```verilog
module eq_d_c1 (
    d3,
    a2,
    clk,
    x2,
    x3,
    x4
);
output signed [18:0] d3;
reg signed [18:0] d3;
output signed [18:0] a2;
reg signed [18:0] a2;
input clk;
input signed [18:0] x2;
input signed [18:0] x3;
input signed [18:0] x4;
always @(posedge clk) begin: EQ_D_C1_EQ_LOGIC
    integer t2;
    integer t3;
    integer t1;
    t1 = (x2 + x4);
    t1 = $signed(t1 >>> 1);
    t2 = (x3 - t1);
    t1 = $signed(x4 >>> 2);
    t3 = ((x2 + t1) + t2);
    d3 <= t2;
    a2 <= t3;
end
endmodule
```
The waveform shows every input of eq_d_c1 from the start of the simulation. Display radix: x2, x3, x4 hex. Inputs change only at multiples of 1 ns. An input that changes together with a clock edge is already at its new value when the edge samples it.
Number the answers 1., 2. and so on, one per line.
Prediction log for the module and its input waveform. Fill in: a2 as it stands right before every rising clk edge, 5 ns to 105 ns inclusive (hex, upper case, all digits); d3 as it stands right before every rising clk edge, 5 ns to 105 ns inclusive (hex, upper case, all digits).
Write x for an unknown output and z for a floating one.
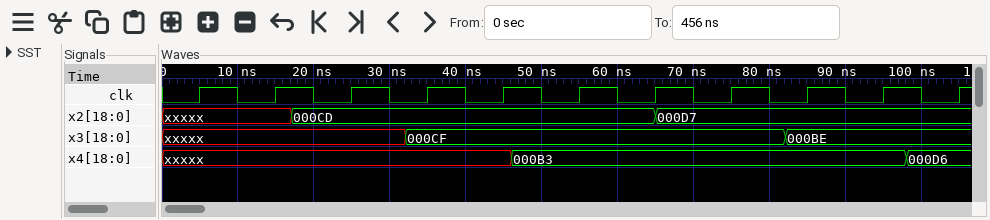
1. x, x, x, x, x, x, 00108, 0010D, 0010D, 000FC, 000FC
2. x, x, x, x, x, x, 0000F, 0000A, 0000A, 7FFF9, 7FFF9
